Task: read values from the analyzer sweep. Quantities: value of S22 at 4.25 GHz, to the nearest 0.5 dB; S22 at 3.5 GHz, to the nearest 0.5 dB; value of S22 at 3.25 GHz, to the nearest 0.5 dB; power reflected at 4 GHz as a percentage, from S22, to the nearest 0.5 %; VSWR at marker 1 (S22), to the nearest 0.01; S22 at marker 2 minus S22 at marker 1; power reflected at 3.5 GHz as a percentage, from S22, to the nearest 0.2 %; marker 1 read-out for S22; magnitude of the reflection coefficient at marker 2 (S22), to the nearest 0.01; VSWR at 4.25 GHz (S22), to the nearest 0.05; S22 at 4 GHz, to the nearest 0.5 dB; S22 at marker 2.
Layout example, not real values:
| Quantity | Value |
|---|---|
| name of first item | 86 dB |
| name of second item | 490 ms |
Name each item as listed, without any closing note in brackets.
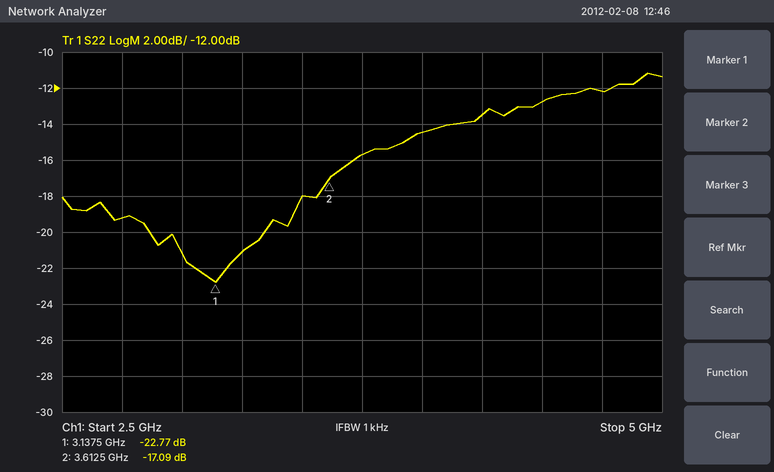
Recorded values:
| Quantity | Value |
|---|---|
| value of S22 at 4.25 GHz, to the nearest 0.5 dB | -13.5 dB |
| S22 at 3.5 GHz, to the nearest 0.5 dB | -18.0 dB |
| value of S22 at 3.25 GHz, to the nearest 0.5 dB | -21.0 dB |
| power reflected at 4 GHz as a percentage, from S22, to the nearest 0.5 % | 3.5 % |
| VSWR at marker 1 (S22), to the nearest 0.01 | 1.16 |
| S22 at marker 2 minus S22 at marker 1 | 5.68 dB |
| power reflected at 3.5 GHz as a percentage, from S22, to the nearest 0.2 % | 1.6 % |
| marker 1 read-out for S22 | -22.77 dB |
| magnitude of the reflection coefficient at marker 2 (S22), to the nearest 0.01 | 0.14 |
| VSWR at 4.25 GHz (S22), to the nearest 0.05 | 1.55 |
| S22 at 4 GHz, to the nearest 0.5 dB | -14.5 dB |
| S22 at marker 2 | -17.09 dB |
